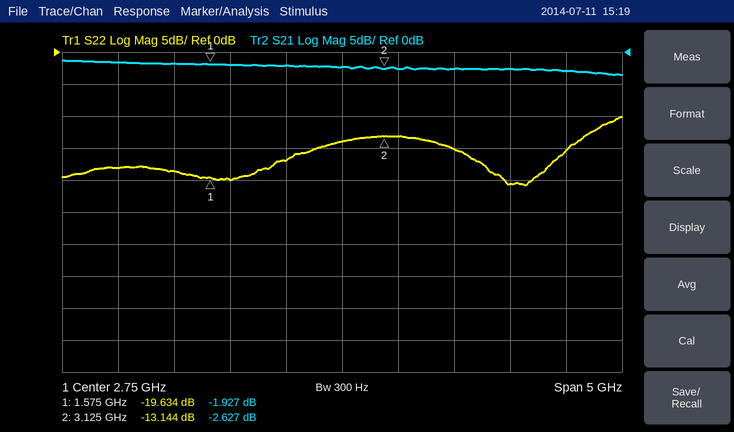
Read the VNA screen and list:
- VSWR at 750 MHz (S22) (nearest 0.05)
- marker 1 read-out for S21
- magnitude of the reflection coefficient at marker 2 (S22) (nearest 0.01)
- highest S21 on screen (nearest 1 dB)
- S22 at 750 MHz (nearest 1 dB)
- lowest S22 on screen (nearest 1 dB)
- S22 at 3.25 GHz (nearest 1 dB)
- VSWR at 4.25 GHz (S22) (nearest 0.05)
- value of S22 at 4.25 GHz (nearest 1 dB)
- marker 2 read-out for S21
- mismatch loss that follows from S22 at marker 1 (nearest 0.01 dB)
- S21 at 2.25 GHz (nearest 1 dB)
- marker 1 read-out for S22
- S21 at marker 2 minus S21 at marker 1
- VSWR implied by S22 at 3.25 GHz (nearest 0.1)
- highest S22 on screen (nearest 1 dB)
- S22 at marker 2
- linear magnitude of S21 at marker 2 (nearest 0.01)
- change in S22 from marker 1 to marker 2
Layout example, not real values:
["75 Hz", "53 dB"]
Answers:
["1.30", "-1.927 dB", "0.22", "-1 dB", "-18 dB", "-21 dB", "-13 dB", "1.20", "-21 dB", "-2.627 dB", "0.05 dB", "-2 dB", "-19.634 dB", "-0.700 dB", "1.6", "-10 dB", "-13.144 dB", "0.74", "6.490 dB"]
